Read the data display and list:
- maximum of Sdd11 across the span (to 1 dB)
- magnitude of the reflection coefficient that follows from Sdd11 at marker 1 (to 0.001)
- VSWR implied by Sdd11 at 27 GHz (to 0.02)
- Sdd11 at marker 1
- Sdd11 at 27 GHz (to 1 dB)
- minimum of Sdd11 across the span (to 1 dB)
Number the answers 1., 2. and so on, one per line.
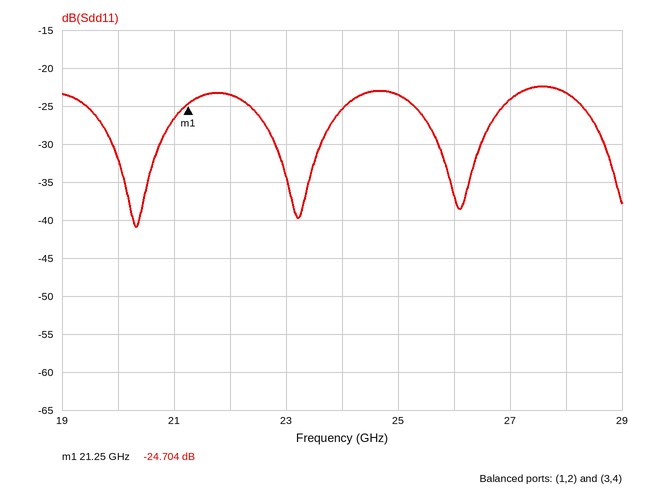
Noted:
1. -22 dB
2. 0.058
3. 1.14
4. -24.704 dB
5. -24 dB
6. -41 dB
